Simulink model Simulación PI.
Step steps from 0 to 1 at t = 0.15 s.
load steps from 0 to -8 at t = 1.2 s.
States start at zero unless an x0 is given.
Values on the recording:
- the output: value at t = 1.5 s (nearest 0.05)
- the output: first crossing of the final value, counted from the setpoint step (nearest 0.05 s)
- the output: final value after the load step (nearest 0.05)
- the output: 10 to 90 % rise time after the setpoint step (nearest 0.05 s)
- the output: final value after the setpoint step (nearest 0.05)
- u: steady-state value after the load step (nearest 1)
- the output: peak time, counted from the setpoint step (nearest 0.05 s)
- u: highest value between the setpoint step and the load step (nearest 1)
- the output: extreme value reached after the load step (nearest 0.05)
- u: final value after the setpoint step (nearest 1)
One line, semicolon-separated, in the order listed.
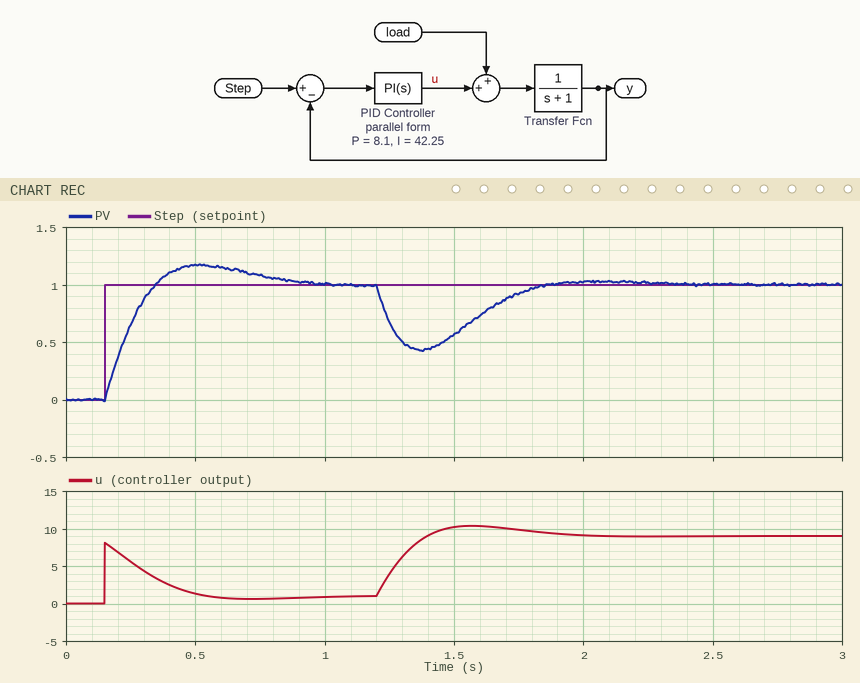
0.55; 0.20 s; 1.00; 0.15 s; 1.00; 9; 0.35 s; 8; 0.45; 1
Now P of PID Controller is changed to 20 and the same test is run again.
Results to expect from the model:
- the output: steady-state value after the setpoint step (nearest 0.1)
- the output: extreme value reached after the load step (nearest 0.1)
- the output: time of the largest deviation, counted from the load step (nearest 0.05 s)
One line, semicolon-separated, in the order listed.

1.0; 0.7; 0.15 s
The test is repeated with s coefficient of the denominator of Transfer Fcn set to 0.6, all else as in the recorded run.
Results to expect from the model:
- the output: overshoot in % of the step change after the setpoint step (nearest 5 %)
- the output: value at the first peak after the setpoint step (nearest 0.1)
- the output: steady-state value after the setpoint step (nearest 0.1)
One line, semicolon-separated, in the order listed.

10 %; 1.1; 1.0
